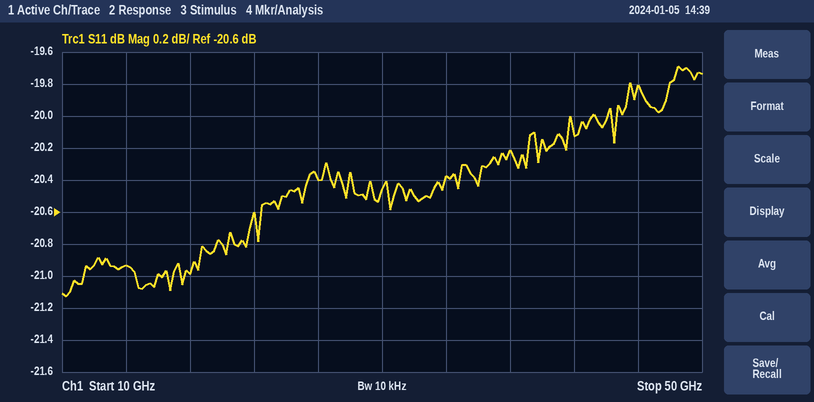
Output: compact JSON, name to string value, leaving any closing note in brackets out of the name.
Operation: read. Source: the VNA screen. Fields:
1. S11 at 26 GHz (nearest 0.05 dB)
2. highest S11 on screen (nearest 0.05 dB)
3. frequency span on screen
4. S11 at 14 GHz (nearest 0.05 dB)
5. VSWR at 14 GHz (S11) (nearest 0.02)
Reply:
{"S11 at 26 GHz": "-20.40 dB", "highest S11 on screen": "-19.70 dB", "frequency span on screen": "40 GHz", "S11 at 14 GHz": "-20.95 dB", "VSWR at 14 GHz (S11)": "1.20"}
